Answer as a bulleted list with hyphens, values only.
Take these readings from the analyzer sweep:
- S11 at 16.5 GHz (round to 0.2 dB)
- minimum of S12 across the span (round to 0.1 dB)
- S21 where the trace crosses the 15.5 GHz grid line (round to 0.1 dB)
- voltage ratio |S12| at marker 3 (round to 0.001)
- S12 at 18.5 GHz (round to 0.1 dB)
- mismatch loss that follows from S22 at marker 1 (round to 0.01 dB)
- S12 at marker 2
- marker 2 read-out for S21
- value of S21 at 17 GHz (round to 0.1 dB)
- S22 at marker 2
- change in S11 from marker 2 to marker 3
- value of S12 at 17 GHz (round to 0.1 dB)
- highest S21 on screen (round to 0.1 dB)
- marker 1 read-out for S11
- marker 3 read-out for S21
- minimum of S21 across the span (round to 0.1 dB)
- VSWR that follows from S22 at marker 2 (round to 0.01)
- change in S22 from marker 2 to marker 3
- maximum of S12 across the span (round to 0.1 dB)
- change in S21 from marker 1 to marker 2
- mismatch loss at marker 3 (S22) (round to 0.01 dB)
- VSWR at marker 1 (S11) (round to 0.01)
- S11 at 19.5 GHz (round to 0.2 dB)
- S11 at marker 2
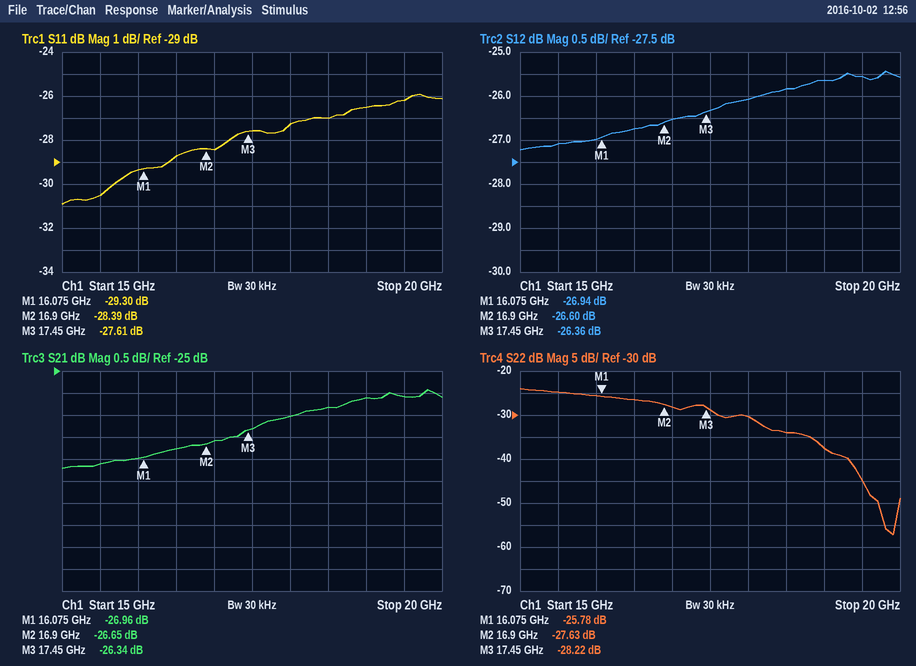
- -28.8 dB
- -27.2 dB
- -27.1 dB
- 0.048
- -25.8 dB
- 0.01 dB
- -26.60 dB
- -26.65 dB
- -26.6 dB
- -27.63 dB
- 0.78 dB
- -26.5 dB
- -25.4 dB
- -29.30 dB
- -26.34 dB
- -27.2 dB
- 1.09
- -0.59 dB
- -25.4 dB
- 0.31 dB
- 0.01 dB
- 1.07
- -26.2 dB
- -28.39 dB
